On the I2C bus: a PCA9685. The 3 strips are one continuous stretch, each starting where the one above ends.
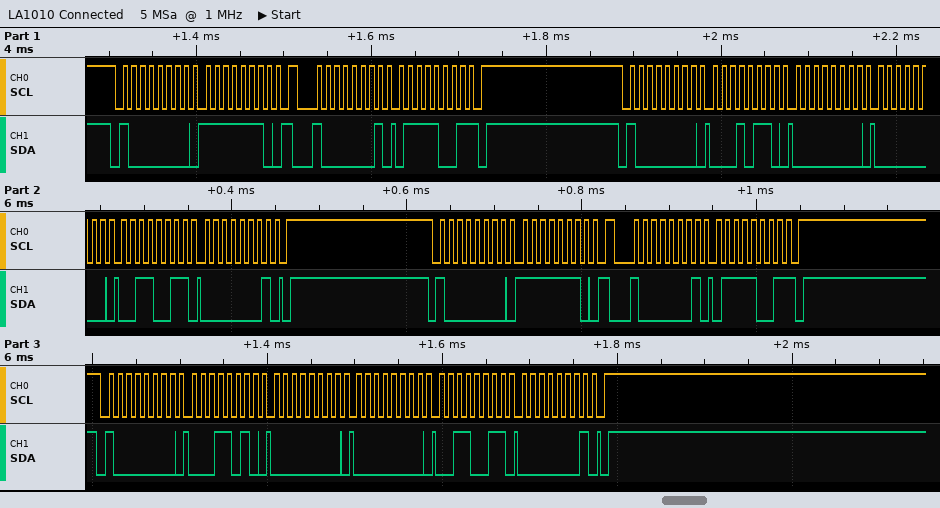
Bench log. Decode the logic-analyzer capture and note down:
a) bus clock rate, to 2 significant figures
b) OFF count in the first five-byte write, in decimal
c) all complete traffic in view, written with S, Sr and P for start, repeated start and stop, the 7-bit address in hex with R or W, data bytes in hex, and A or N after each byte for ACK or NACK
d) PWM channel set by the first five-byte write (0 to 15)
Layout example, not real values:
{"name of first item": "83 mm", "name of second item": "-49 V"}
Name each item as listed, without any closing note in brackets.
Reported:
{"bus clock rate, to 2 significant figures": "100 kHz", "OFF count in the first five-byte write, in decimal": "307", "all complete traffic in view, written with S, Sr and P for start, repeated start and stop, the 7-bit address in hex with R or W, data bytes in hex, and A or N after each byte for ACK or NACK": "S 40W A FE A Sr 40R A 79 N P S 40W A 16 A 00 A 00 A 33 A 01 A P S 40W A FE A Sr 40R A 79 N P S 40W A 1A A 00 A 00 A 33 A 01 A P", "PWM channel set by the first five-byte write": "4"}
